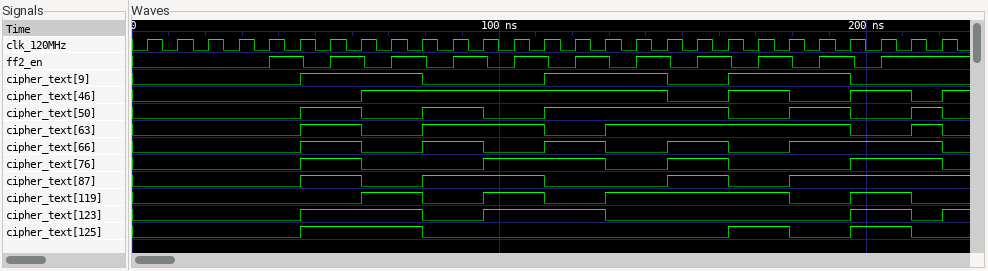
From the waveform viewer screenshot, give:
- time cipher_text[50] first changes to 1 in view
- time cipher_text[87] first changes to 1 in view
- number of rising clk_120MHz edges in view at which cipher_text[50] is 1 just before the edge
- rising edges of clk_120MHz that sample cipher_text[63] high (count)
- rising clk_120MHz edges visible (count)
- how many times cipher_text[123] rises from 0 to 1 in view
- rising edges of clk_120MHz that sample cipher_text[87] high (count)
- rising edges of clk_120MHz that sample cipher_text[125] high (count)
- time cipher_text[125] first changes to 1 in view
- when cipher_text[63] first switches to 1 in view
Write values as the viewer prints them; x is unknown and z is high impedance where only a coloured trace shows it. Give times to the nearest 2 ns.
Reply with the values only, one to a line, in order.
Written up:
46 ns
46 ns
13
15
27
4
13
8
46 ns
46 ns
